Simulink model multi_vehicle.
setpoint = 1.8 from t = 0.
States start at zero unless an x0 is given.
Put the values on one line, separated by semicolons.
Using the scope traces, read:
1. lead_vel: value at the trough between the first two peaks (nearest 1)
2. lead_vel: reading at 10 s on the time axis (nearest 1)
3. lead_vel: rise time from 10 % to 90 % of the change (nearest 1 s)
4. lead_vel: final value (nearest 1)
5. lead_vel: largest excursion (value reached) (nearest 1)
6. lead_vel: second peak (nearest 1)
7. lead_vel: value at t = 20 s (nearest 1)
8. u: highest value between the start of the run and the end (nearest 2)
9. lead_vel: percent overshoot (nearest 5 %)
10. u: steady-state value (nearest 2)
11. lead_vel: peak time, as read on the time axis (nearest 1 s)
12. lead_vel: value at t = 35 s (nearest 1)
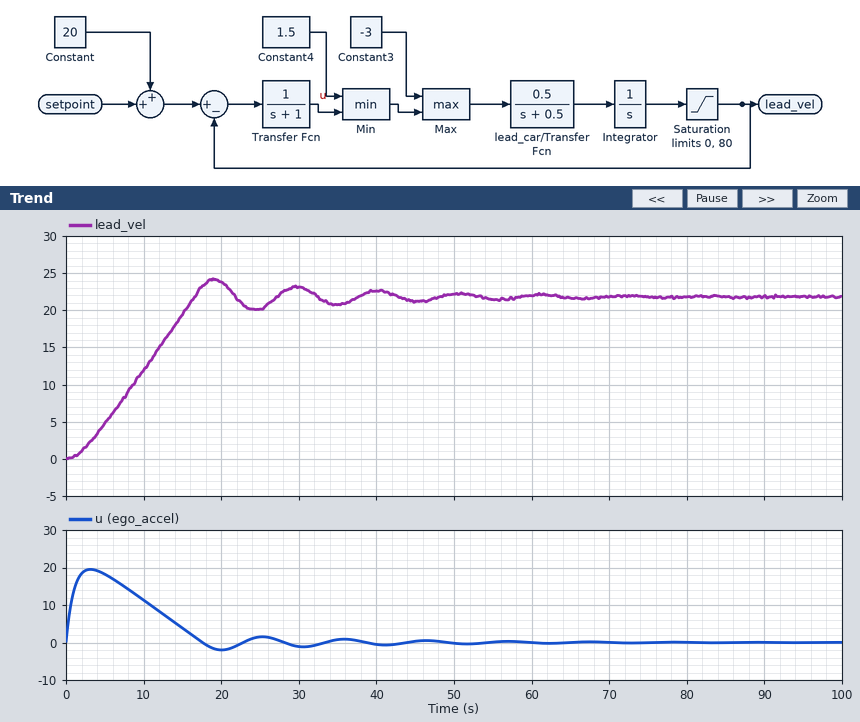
20; 12; 12 s; 22; 24; 23; 24; 20; 10 %; 0; 19 s; 21
